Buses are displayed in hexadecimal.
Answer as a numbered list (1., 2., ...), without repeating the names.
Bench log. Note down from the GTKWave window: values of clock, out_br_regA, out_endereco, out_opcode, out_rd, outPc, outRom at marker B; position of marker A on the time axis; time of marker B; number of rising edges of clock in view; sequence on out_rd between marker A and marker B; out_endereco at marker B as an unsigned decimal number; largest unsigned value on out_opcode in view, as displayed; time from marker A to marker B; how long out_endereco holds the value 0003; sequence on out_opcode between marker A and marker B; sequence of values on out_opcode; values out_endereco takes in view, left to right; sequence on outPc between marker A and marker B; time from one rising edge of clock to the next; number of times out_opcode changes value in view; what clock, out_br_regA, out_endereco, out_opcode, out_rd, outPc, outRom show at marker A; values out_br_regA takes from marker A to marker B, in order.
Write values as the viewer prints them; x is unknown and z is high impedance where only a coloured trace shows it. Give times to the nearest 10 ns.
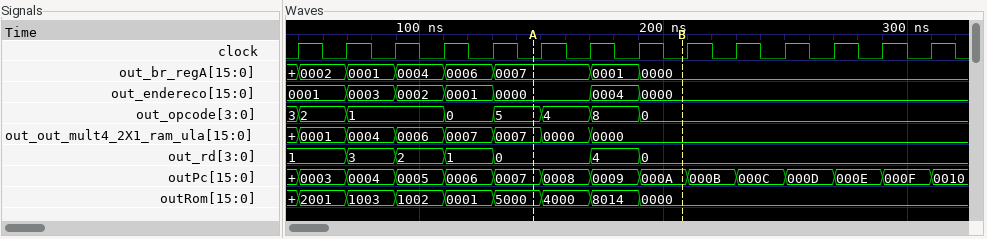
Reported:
1. clock=0, out_br_regA=0000, out_endereco=0000, out_opcode=0, out_rd=0, outPc=000A, outRom=0000
2. 150 ns
3. 210 ns
4. 14
5. 0, 4, 0
6. 0
7. 8
8. 60 ns
9. 20 ns
10. 5, 4, 8, 0
11. 3, 2, 1, 0, 5, 4, 8, 0
12. 0001, 0003, 0002, 0001, 0000, 0004, 0000
13. 0007, 0008, 0009, 000A
14. 20 ns
15. 7
16. clock=0, out_br_regA=0007, out_endereco=0000, out_opcode=5, out_rd=0, outPc=0007, outRom=5000
17. 0007, 0001, 0000
